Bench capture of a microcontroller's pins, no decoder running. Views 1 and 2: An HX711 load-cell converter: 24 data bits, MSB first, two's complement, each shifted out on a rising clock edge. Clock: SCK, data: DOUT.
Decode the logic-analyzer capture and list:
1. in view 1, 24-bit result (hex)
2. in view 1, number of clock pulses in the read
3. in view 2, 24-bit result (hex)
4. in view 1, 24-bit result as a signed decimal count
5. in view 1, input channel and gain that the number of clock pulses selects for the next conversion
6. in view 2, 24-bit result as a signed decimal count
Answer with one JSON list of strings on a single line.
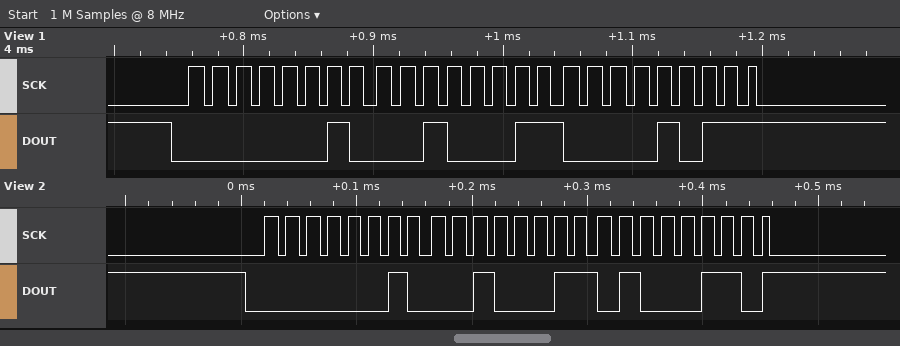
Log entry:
["0x02230B", "25", "0x022346", "140043", "channel A, gain 128", "140102"]
